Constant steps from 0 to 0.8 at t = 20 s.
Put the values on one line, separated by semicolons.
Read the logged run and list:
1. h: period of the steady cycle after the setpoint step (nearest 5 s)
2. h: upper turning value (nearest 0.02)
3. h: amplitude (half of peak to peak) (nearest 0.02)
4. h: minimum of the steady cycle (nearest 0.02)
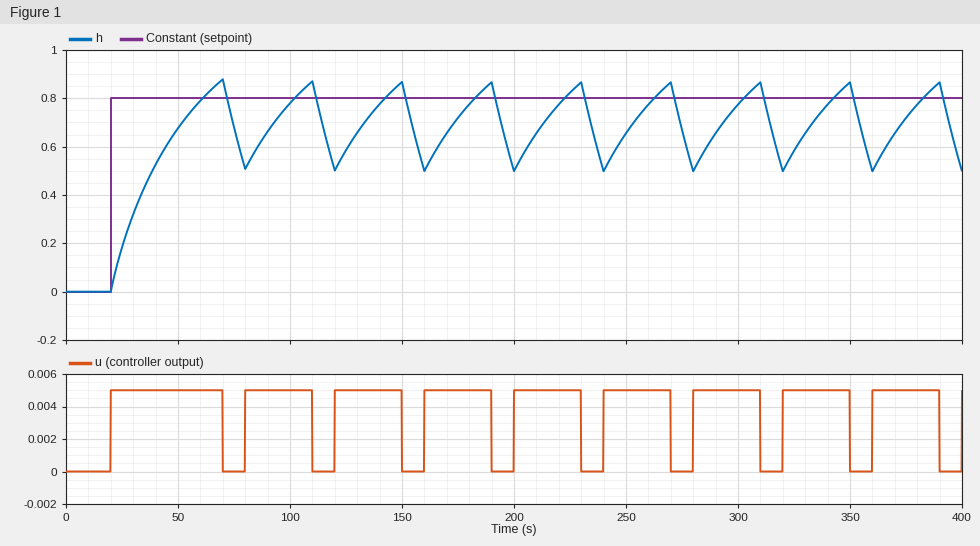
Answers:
40 s; 0.86; 0.18; 0.50
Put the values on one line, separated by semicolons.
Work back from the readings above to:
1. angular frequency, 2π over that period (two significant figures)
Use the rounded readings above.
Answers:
0.16 rad/s
